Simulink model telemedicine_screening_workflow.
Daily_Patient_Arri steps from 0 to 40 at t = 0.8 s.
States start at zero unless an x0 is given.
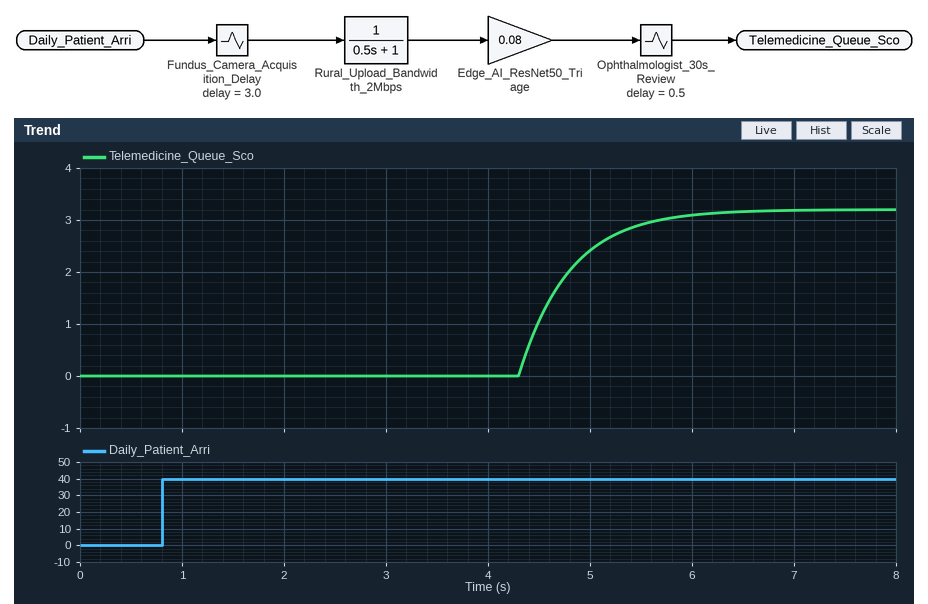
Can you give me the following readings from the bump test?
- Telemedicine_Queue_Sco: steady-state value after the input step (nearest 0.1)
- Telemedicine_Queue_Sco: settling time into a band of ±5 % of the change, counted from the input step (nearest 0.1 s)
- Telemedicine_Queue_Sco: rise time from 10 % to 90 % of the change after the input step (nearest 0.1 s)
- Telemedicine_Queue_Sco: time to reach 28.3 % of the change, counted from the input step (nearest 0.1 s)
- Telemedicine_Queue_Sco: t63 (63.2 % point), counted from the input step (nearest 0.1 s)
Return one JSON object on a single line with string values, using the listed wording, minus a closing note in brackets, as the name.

{"Telemedicine_Queue_Sco: steady-state value after the input step": "3.2", "Telemedicine_Queue_Sco: settling time into a band of ±5 % of the change, counted from the input step": "5.0 s", "Telemedicine_Queue_Sco: rise time from 10 % to 90 % of the change after the input step": "1.1 s", "Telemedicine_Queue_Sco: time to reach 28.3 % of the change, counted from the input step": "3.7 s", "Telemedicine_Queue_Sco: t63 (63.2 % point), counted from the input step": "4.0 s"}
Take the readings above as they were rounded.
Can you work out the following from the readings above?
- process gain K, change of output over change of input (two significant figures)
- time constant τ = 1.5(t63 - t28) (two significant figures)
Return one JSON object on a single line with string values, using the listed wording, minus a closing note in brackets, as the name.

{"process gain K, change of output over change of input": "0.080", "time constant τ = 1.5(t63 - t28)": "0.45 s"}
